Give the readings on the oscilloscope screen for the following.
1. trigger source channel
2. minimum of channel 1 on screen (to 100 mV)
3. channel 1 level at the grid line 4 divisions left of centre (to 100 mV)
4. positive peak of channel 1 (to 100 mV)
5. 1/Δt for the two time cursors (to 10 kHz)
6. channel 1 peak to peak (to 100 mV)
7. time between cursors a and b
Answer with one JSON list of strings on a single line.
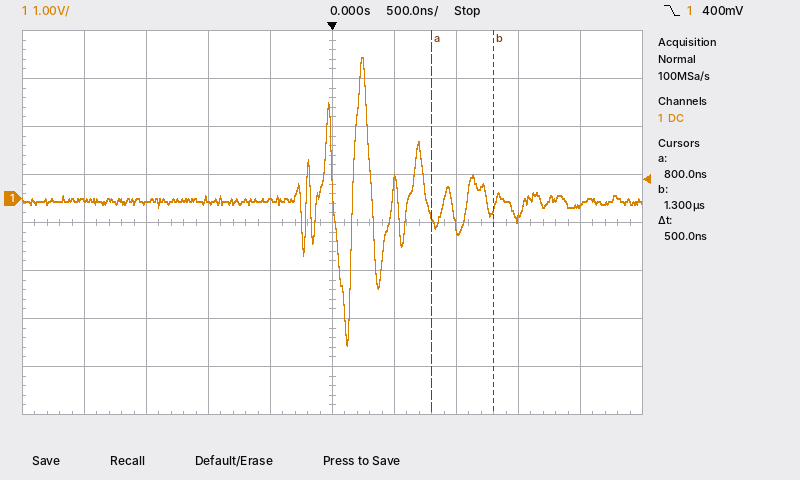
["channel 1", "-3.1 V", "0.0 V", "2.9 V", "2.00 MHz", "6.0 V", "500 ns"]
